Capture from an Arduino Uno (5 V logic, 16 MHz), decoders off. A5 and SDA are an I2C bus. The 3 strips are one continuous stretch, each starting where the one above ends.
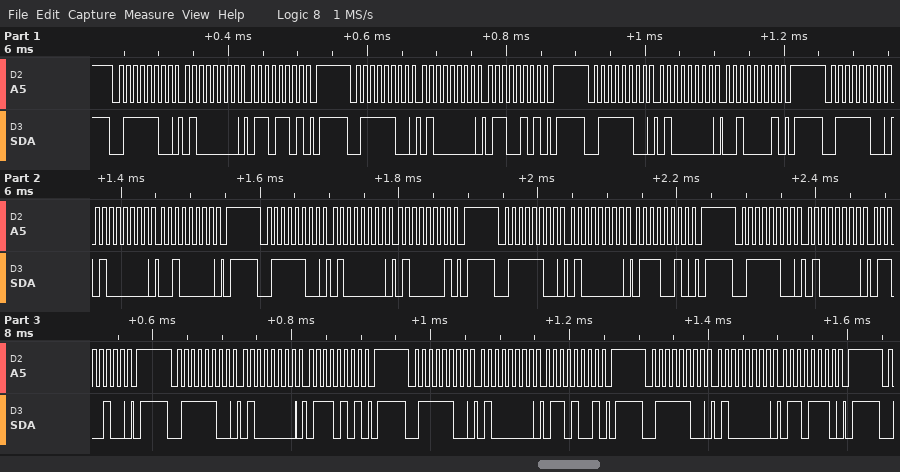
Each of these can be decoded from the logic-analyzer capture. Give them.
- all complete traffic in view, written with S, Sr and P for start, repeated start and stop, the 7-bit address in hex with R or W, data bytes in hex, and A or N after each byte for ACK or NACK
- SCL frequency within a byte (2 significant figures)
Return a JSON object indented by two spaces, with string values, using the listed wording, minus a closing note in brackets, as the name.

{
  "all complete traffic in view, written with S, Sr and P for start, repeated start and stop, the 7-bit address in hex with R or W, data bytes in hex, and A or N after each byte for ACK or NACK": "S 3EW A 40 A 6D A P S 3EW A 40 A 65 A P S 3EW A 40 A 21 A P S 3EW A 40 A 20 A P S 3EW A 40 A 41 A P S 3EW A 40 A 72 A P S 3EW A 40 A 64 A P S 3EW A 40 A 75 A P S 3EW A 40 A 69 A P S 3EW A 40 A 6E A P",
  "SCL frequency within a byte": "100 kHz"
}
